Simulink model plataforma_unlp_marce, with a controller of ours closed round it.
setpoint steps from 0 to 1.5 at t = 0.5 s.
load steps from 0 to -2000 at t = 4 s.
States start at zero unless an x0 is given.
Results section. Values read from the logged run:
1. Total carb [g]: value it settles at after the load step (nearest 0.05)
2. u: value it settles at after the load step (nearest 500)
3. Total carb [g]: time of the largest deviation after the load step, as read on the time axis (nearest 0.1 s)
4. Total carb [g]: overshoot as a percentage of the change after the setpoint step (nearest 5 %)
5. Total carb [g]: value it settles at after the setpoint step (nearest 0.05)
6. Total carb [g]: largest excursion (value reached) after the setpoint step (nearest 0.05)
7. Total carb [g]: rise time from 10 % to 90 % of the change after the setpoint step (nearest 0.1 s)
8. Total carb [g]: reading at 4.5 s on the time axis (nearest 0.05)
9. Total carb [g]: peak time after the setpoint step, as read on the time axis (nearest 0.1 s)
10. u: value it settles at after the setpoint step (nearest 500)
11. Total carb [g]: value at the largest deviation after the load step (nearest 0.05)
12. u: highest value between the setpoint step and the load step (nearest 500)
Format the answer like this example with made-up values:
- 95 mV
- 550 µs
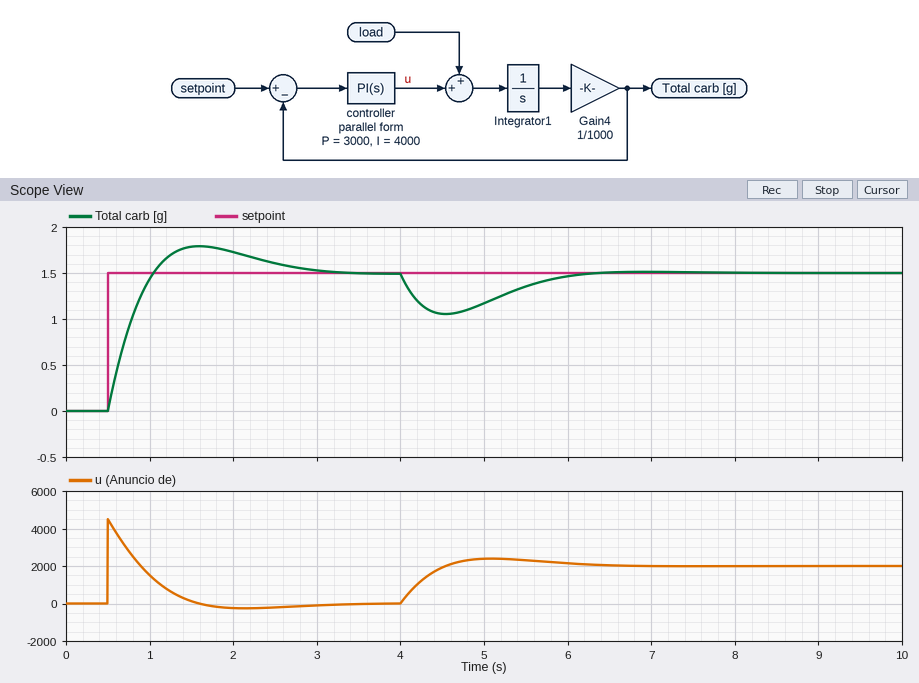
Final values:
- 1.50
- 2000
- 4.5 s
- 20 %
- 1.50
- 1.80
- 0.4 s
- 1.05
- 1.6 s
- 0
- 1.05
- 4500
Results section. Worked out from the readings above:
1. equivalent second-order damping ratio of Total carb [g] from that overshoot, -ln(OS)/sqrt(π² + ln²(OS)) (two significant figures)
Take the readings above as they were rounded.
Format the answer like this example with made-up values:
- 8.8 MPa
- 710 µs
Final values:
- 0.46
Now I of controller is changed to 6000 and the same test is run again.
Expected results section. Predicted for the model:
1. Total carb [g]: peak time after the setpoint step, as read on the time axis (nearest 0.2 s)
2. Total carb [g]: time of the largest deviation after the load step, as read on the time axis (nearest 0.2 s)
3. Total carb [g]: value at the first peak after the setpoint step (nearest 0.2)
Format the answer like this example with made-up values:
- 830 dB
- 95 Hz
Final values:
- 1.4 s
- 4.4 s
- 1.8
